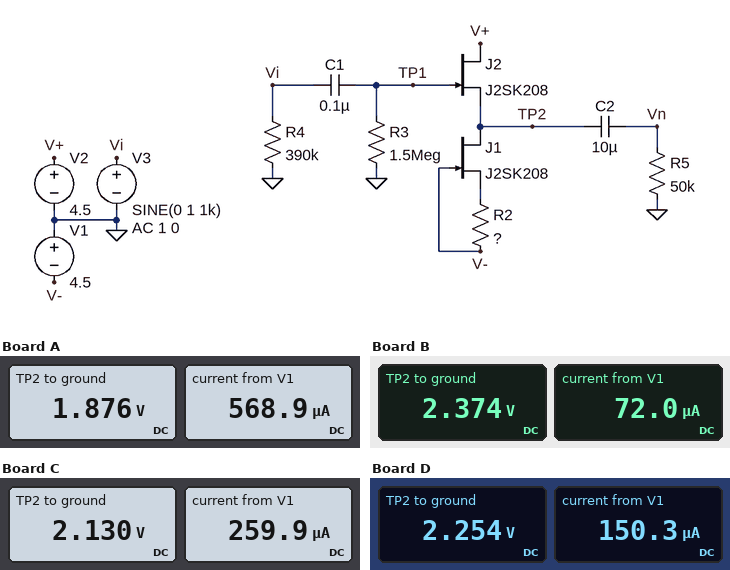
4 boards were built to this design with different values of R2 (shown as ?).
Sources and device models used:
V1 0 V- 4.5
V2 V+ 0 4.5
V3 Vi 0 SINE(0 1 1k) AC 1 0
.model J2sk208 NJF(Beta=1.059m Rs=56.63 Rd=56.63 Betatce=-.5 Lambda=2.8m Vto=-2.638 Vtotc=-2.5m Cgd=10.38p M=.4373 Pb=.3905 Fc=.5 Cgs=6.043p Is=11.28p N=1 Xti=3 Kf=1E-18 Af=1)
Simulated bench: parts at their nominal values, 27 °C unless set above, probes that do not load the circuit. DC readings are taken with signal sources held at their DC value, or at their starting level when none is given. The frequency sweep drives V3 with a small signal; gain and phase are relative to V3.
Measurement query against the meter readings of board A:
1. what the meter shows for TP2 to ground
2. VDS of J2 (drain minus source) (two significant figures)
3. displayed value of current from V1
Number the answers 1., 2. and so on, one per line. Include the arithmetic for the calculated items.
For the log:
1. 1.876 V
2. 4.5 V - 1.876 V = 2.6 V
3. 568.9 µA
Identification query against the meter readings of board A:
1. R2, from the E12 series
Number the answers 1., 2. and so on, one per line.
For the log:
1. 3.3 kΩ
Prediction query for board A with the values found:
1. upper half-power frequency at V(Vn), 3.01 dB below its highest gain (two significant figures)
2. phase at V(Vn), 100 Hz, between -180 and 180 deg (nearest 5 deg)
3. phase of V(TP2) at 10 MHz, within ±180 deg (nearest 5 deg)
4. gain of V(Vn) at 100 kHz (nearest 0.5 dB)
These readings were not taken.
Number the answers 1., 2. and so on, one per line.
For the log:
1. 66 MHz
2. 0 deg
3. -5 deg
4. 0 dB
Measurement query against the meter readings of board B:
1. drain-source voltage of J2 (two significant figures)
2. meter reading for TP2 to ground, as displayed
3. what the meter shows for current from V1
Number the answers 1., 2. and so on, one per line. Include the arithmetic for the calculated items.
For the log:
1. 4.5 V - 2.374 V = 2.1 V
2. 2.374 V
3. 72.0 µA
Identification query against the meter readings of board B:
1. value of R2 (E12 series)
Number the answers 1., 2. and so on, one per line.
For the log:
1. 33 kΩ
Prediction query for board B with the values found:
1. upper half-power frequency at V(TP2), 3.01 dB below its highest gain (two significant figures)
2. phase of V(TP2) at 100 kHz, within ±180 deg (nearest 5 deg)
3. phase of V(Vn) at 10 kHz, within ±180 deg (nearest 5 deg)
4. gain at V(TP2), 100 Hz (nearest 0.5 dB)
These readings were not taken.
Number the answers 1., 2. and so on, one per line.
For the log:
1. 27 MHz
2. 0 deg
3. 0 deg
4. -0.5 dB
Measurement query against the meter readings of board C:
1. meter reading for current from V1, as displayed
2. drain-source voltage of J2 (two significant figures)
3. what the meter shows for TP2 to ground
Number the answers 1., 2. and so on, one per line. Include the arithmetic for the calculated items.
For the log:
1. 259.9 µA
2. 4.5 V - 2.13 V = 2.4 V
3. 2.130 V
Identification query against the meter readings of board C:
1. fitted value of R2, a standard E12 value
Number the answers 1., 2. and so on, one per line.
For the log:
1. 8.2 kΩ
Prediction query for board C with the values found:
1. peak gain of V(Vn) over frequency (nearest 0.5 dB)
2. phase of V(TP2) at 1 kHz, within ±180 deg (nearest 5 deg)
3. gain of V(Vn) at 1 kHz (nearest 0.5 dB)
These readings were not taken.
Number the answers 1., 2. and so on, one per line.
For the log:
1. 0 dB
2. 0 deg
3. 0 dB
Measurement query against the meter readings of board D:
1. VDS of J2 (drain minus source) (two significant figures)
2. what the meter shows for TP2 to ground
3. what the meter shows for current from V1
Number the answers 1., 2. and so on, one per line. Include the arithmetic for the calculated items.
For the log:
1. 4.5 V - 2.254 V = 2.2 V
2. 2.254 V
3. 150.3 µA
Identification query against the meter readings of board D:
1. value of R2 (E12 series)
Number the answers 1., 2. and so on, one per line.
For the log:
1. 15 kΩ
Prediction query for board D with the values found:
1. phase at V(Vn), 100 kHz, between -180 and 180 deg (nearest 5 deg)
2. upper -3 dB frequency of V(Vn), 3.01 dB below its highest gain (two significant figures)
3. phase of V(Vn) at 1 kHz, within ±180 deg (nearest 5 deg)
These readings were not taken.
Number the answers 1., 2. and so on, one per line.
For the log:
1. 0 deg
2. 37 MHz
3. 0 deg
